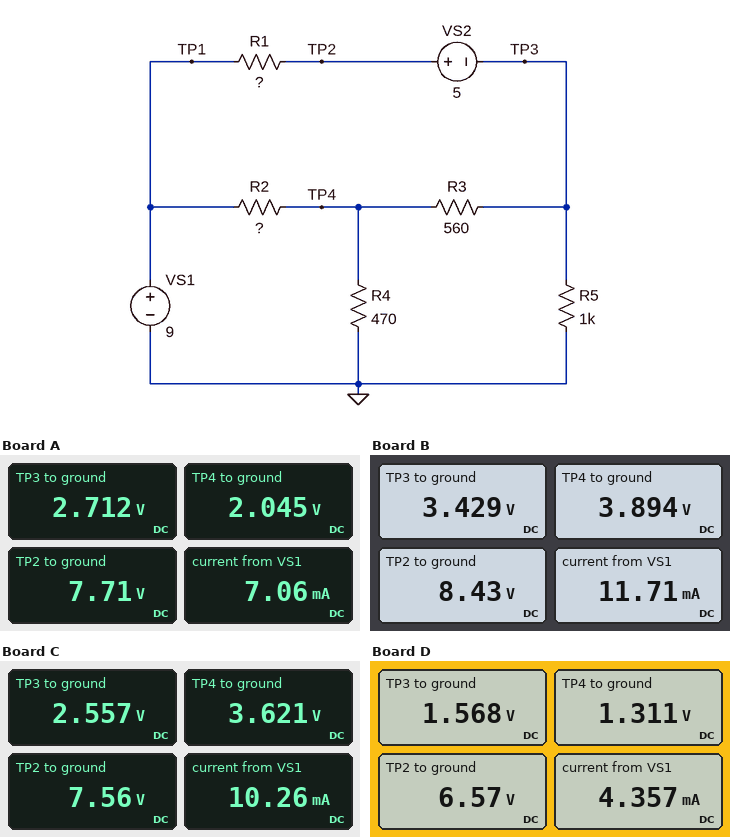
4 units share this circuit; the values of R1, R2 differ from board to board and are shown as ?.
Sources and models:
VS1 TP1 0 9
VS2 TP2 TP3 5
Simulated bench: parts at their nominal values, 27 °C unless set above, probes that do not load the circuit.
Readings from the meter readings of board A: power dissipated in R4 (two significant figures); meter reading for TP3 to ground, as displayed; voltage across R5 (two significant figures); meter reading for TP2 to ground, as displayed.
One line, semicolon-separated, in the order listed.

8.9 mW; 2.712 V; 2.7 V; 7.71 V
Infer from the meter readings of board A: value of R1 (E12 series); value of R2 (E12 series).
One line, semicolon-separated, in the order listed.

330 Ω; 2.2 kΩ
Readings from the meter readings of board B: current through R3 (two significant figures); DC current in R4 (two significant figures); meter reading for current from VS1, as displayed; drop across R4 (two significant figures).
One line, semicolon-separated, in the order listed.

830 µA; 8.3 mA; 11.71 mA; 3.9 V
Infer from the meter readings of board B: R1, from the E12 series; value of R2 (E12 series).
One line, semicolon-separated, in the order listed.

220 Ω; 560 Ω
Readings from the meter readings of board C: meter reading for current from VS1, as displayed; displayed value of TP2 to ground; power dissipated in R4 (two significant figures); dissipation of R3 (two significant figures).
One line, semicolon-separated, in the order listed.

10.26 mA; 7.56 V; 28 mW; 2.0 mW
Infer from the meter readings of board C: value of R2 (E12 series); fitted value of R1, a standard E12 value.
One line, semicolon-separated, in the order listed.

560 Ω; 2.2 kΩ
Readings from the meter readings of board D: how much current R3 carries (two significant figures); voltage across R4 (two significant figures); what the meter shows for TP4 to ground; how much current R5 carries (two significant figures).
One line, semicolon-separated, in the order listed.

460 µA; 1.3 V; 1.311 V; 1.6 mA
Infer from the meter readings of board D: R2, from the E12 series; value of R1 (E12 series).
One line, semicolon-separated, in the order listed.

3.3 kΩ; 1.2 kΩ
